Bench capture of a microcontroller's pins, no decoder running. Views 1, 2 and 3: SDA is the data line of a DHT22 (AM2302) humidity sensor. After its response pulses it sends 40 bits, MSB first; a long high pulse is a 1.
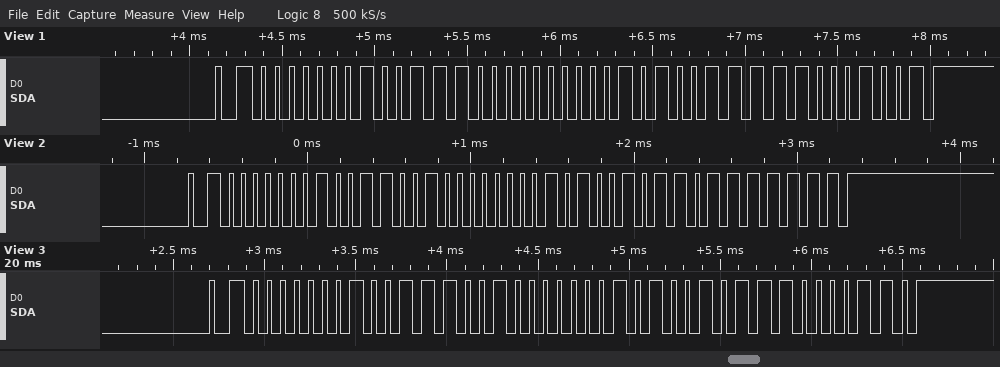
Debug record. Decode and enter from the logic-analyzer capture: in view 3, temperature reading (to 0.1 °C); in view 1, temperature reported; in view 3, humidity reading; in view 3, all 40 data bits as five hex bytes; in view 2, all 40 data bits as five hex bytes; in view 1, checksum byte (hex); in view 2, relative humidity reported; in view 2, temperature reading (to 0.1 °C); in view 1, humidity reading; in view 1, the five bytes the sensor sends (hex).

33.1 °C
33.5 °C
31.3 %
01 39 01 4B 86
01 32 01 4B 7F
0x89
30.6 %
33.1 °C
31.2 %
01 38 01 4F 89
